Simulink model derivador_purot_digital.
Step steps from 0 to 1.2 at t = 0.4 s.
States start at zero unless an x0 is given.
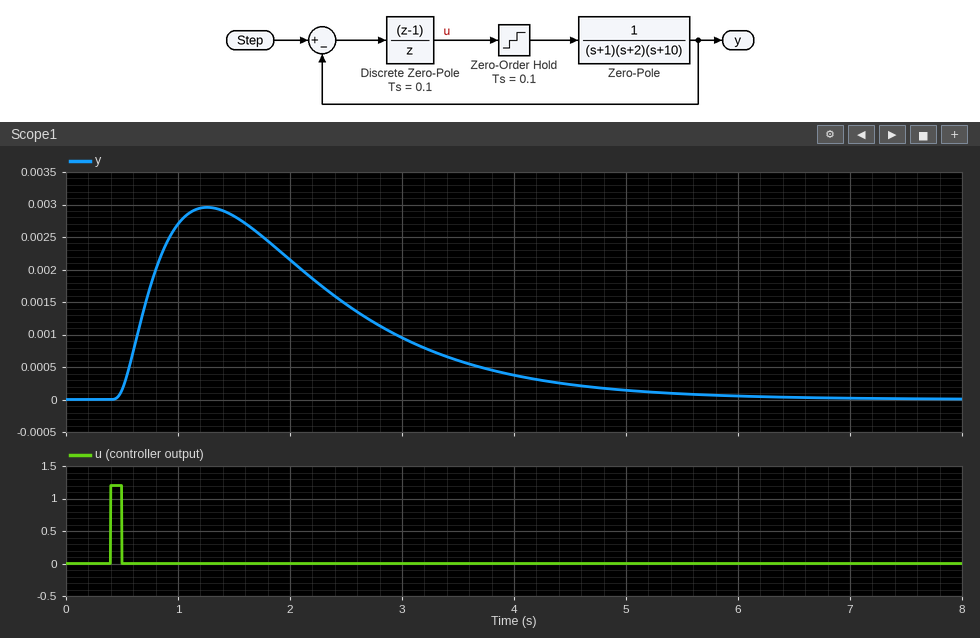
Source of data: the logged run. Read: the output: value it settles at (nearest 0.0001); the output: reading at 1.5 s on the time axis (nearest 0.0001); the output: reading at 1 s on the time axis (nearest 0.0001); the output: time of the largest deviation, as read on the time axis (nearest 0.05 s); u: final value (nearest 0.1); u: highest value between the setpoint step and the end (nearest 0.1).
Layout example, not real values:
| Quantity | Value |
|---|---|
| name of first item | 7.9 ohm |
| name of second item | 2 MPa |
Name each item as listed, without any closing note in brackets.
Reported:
| Quantity | Value |
|---|---|
| the output: value it settles at | 0.0000 |
| the output: reading at 1.5 s on the time axis | 0.0028 |
| the output: reading at 1 s on the time axis | 0.0027 |
| the output: time of the largest deviation, as read on the time axis | 1.25 s |
| u: final value | 0.0 |
| u: highest value between the setpoint step and the end | 1.2 |
